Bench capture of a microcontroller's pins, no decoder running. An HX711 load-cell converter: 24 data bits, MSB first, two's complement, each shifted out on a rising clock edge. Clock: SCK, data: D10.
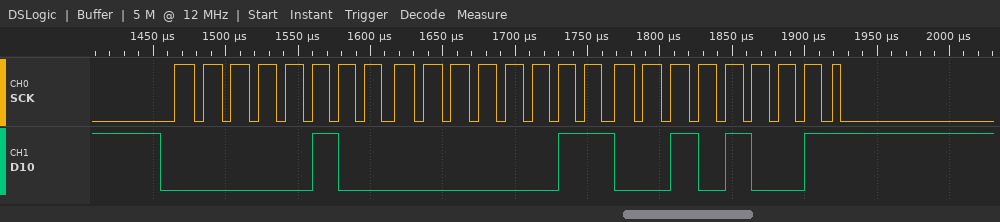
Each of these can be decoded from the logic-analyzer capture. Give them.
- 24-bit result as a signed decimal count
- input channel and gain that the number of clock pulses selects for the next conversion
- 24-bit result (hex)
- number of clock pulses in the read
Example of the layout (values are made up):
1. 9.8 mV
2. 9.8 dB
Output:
1. 262953
2. channel A, gain 128
3. 0x040329
4. 25
